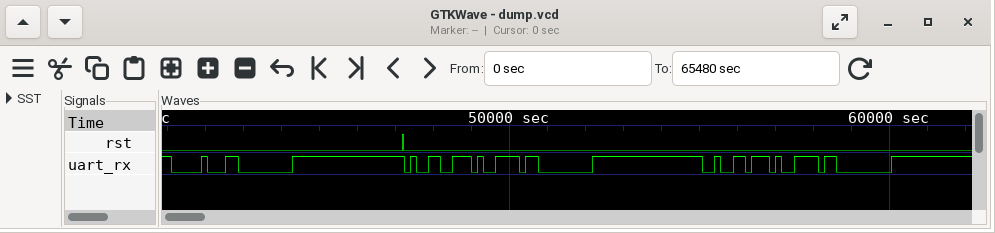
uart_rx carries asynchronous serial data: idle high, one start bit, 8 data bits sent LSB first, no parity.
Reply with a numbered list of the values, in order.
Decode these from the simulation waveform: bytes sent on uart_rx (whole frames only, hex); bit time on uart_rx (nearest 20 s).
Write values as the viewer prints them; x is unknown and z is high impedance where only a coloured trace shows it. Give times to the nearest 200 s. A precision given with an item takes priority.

1. 10, 00, 99, 79, 00, B2, 79, 00
2. 160 s
